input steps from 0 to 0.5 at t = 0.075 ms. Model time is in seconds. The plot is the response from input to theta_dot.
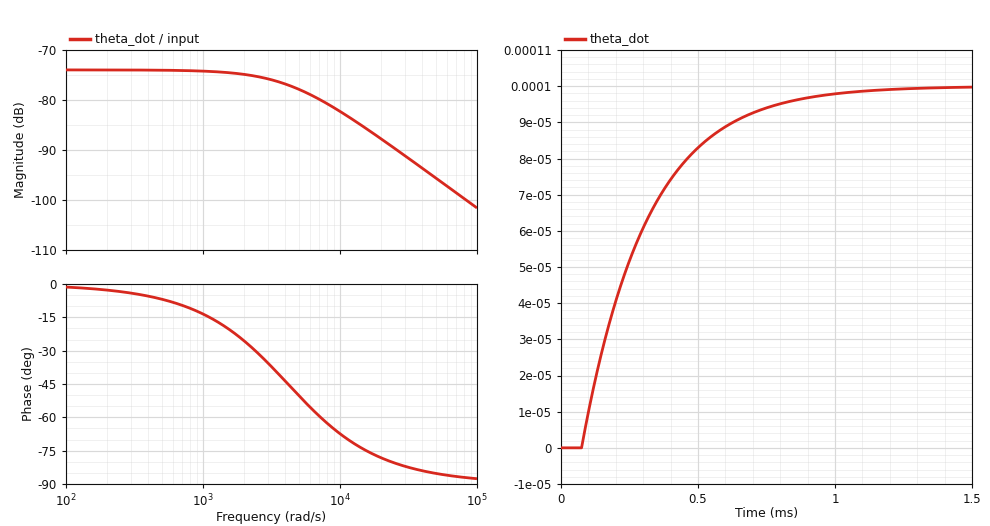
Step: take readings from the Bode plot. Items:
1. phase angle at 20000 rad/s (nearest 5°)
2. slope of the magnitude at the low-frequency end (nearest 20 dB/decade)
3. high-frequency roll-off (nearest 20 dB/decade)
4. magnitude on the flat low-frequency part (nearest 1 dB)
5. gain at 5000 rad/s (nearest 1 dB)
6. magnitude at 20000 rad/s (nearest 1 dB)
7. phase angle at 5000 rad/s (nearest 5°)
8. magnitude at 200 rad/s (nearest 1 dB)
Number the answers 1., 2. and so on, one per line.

1. -80°
2. 0 dB/decade
3. -20 dB/decade
4. -74 dB
5. -78 dB
6. -88 dB
7. -50°
8. -74 dB
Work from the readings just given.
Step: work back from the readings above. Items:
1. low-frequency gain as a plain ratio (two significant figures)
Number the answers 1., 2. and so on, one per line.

1. 0.00020
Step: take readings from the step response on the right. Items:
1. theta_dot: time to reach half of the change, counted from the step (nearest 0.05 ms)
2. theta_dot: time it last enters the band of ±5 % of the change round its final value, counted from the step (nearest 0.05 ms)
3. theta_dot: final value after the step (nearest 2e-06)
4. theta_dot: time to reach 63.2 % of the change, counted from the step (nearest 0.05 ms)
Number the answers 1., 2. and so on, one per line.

1. 0.15 ms
2. 0.70 ms
3. 0.000100
4. 0.25 ms
